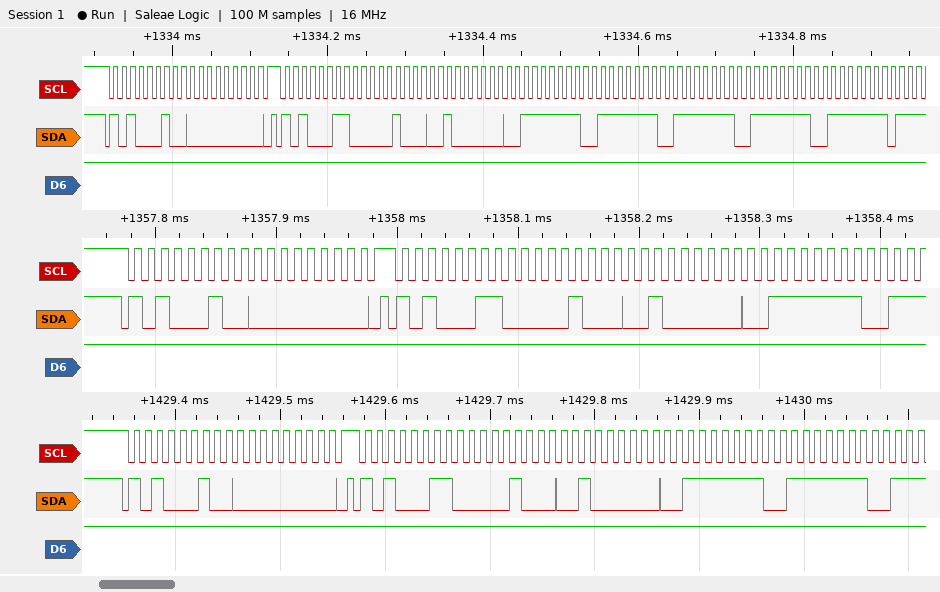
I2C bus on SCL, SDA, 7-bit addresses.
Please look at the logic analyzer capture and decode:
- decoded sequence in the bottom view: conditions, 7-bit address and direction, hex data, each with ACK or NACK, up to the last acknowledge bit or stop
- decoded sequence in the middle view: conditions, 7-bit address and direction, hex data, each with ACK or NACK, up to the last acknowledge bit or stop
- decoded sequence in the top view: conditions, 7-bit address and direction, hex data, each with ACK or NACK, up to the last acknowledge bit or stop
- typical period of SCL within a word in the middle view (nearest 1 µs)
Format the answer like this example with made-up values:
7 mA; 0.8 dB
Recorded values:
start, address 51 write ACK, 00 ACK, stop, start, address 51 read ACK, 08 ACK, 40 ACK, 7F ACK, 7F ACK; start, address 51 write ACK, 00 ACK, stop, start, address 51 read ACK, 08 ACK, 40 ACK, 7F ACK; start, address 51 write ACK, 00 ACK, stop, start, address 51 read ACK, 08 ACK, 40 ACK, 7F ACK, 7F ACK, 7F ACK, 7F ACK, 7F ACK; 11 µs
